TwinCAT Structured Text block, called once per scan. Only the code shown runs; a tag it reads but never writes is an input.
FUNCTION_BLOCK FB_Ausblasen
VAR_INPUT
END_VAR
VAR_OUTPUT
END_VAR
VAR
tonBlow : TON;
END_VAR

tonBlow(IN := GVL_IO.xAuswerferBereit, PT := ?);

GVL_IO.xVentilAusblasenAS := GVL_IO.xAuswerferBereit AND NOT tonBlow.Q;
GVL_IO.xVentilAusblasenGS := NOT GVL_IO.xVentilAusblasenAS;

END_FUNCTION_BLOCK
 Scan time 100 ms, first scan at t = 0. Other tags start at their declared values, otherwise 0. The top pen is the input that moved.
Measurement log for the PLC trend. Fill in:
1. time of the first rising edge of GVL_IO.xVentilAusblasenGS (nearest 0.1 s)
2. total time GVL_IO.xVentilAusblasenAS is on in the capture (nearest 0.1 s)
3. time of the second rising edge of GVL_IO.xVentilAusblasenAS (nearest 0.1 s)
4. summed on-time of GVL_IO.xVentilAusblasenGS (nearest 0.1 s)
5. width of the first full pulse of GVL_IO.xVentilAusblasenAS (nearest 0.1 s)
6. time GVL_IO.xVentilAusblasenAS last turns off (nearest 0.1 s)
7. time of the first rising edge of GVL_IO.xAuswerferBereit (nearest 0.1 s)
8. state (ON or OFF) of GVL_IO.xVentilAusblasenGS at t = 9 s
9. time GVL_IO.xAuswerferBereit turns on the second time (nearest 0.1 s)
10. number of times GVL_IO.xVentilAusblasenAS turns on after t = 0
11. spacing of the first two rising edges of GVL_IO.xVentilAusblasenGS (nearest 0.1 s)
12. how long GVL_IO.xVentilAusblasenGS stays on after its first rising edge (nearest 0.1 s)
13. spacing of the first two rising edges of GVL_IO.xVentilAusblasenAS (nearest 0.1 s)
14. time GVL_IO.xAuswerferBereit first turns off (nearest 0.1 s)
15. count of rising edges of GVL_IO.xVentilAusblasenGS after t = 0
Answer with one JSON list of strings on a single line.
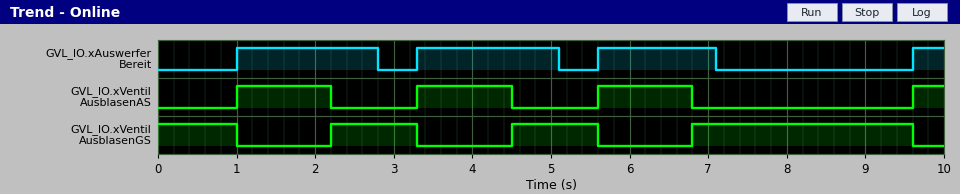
["2.2 s", "4.0 s", "3.3 s", "6.0 s", "1.2 s", "6.8 s", "1.0 s", "ON", "3.3 s", "4", "2.3 s", "1.1 s", "2.3 s", "2.8 s", "3"]
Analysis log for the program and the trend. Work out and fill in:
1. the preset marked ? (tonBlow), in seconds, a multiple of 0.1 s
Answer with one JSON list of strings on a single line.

["1.2 s"]
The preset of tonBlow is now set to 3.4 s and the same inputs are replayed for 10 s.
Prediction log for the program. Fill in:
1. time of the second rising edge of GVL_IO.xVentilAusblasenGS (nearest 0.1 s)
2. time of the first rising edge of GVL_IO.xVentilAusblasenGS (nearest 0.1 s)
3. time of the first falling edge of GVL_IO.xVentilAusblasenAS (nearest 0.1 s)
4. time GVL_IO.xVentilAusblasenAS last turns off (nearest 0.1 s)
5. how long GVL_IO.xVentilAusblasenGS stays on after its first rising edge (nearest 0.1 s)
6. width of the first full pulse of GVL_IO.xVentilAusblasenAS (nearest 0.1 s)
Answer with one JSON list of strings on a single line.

["5.1 s", "2.8 s", "2.8 s", "7.1 s", "0.5 s", "1.8 s"]
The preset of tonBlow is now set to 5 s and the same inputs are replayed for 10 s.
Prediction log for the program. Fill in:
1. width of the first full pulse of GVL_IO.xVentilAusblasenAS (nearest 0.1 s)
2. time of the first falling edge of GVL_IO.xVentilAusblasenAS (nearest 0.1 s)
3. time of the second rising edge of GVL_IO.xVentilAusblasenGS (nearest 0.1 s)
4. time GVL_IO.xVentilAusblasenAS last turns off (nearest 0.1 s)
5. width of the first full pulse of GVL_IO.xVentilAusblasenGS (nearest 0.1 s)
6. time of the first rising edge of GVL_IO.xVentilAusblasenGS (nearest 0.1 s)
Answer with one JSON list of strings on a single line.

["1.8 s", "2.8 s", "5.1 s", "7.1 s", "0.5 s", "2.8 s"]
